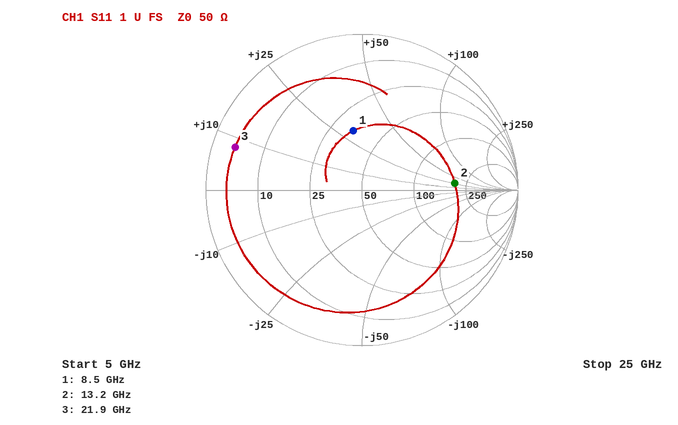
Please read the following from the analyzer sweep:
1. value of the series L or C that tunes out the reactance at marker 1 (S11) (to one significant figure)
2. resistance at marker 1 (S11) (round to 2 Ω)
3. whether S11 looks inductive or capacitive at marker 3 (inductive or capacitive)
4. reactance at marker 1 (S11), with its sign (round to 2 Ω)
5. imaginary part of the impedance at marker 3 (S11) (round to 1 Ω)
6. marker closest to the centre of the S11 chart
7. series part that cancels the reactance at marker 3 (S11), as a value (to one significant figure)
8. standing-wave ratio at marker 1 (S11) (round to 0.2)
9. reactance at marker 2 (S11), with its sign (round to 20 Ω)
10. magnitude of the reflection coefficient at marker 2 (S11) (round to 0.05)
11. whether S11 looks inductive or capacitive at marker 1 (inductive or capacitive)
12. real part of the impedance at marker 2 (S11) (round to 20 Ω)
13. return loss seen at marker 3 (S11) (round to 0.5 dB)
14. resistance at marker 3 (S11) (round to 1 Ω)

600 fF
34 Ω
inductive
+30 Ω
+8 Ω
marker 1
900 fF
2.2
+20 Ω
0.60
inductive
200 Ω
1.5 dB
4 Ω
